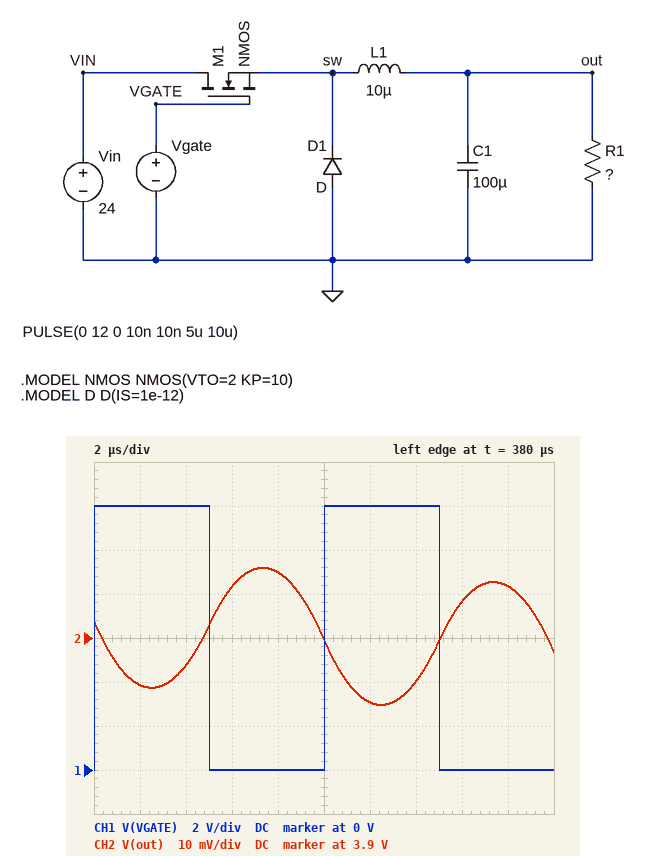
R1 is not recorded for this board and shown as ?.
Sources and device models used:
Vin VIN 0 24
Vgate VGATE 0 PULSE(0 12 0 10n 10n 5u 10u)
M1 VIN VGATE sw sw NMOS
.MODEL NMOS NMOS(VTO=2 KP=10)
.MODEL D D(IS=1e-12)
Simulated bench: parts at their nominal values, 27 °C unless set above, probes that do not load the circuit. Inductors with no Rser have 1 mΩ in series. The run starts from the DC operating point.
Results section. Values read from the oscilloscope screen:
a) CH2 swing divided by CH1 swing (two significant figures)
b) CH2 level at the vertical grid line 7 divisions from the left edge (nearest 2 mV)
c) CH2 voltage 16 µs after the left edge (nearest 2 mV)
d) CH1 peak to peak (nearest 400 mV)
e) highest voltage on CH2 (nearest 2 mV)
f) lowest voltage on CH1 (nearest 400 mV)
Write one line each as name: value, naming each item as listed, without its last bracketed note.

CH2 swing divided by CH1 swing: 0.0026
CH2 level at the vertical grid line 7 divisions from the left edge: 3.890 V
CH2 voltage 16 µs after the left edge: 3.908 V
CH1 peak to peak: 12.0 V
highest voltage on CH2: 3.916 V
lowest voltage on CH1: 0 V
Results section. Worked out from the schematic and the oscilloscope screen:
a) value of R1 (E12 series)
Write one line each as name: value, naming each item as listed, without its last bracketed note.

value of R1: 0.39 Ω
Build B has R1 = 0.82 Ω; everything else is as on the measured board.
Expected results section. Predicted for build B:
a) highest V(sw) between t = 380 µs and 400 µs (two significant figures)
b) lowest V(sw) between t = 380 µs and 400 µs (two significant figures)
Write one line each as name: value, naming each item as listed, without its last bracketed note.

highest V(sw) between t = 380 µs and 400 µs: 9.2 V
lowest V(sw) between t = 380 µs and 400 µs: -760 mV
